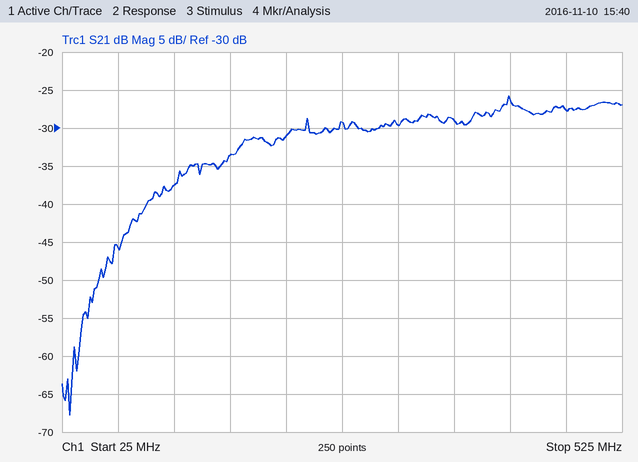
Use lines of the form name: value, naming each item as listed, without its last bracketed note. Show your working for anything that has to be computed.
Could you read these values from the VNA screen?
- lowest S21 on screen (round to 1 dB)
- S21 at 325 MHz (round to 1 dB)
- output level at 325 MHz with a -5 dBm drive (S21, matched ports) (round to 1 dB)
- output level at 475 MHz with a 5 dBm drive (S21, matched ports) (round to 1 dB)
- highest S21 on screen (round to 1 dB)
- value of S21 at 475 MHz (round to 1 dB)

lowest S21 on screen: -68 dB
S21 at 325 MHz: -30 dB
output level at 325 MHz with a -5 dBm drive (S21, matched ports): -5 dBm + (-30 dB) = -35 dBm
output level at 475 MHz with a 5 dBm drive (S21, matched ports): 5 dBm + (-28 dB) = -23 dBm
highest S21 on screen: -26 dB
value of S21 at 475 MHz: -28 dB
